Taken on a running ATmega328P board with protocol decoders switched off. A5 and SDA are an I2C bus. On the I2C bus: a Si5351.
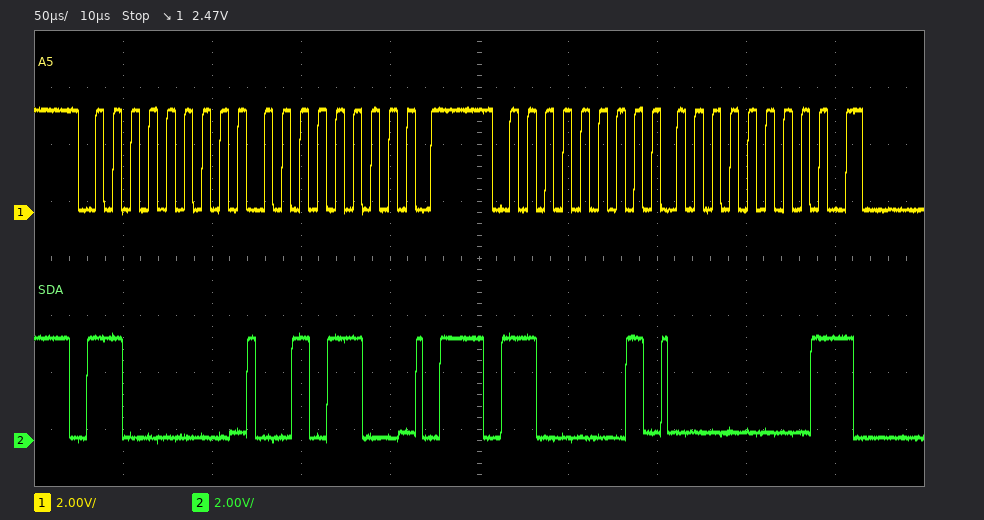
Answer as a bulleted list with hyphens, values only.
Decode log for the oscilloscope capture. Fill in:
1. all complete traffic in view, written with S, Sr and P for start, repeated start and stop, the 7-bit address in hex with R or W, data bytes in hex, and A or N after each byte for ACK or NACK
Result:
- S 60W A 2C A P S 60R A 00 N
